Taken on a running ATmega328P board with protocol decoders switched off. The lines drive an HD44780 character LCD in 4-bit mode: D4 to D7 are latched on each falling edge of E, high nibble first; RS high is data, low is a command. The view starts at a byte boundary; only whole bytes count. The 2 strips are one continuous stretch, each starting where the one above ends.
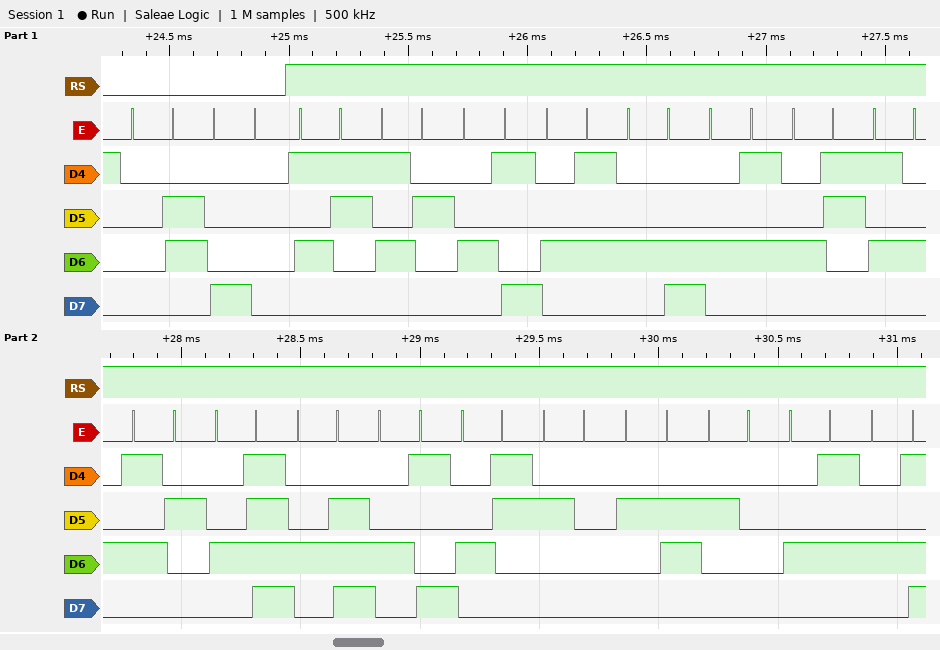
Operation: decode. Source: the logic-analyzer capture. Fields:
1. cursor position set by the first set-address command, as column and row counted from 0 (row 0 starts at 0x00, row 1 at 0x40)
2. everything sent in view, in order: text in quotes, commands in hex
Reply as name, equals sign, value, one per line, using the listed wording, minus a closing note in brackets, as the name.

cursor position set by the first set-address command, as column and row counted from 0 = column 0, row 0
everything sent in view, in order: text in quotes, commands in hex = 0x06 0x80 "SRIELECTRONIC & EM"
